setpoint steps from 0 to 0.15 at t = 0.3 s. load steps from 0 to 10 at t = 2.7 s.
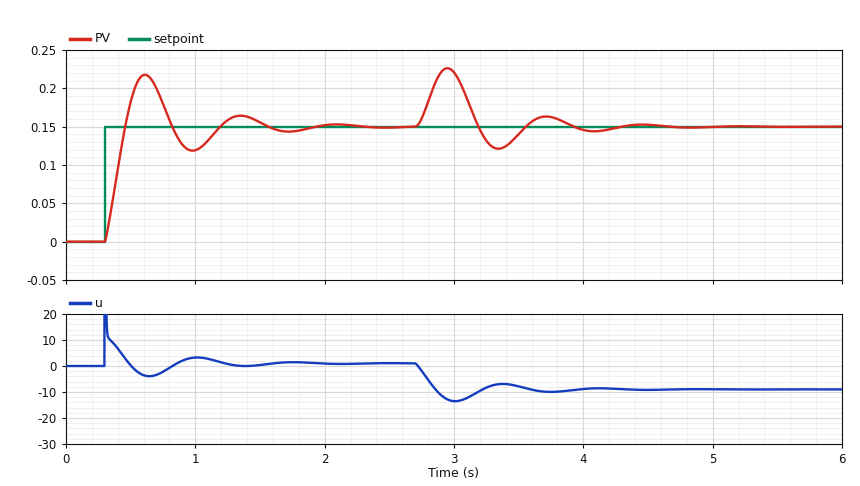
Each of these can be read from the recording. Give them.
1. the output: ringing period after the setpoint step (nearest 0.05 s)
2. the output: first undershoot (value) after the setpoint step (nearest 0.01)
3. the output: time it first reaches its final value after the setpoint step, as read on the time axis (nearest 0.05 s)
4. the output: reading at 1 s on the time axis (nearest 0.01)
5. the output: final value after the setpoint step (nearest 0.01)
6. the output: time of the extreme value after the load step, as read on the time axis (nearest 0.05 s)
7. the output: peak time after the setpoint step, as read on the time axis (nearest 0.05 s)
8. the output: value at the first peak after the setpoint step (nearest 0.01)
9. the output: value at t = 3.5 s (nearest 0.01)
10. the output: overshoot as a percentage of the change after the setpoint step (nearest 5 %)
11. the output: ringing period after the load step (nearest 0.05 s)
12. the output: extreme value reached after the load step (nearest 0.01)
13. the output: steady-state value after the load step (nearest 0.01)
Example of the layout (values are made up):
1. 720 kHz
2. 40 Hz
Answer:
1. 0.75 s
2. 0.12
3. 0.45 s
4. 0.12
5. 0.15
6. 2.95 s
7. 0.60 s
8. 0.22
9. 0.14
10. 45 %
11. 0.75 s
12. 0.23
13. 0.15
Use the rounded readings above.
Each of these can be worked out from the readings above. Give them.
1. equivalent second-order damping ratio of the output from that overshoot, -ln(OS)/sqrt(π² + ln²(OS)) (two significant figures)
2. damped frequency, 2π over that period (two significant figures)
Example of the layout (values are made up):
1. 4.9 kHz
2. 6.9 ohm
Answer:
1. 0.25
2. 8.4 rad/s
